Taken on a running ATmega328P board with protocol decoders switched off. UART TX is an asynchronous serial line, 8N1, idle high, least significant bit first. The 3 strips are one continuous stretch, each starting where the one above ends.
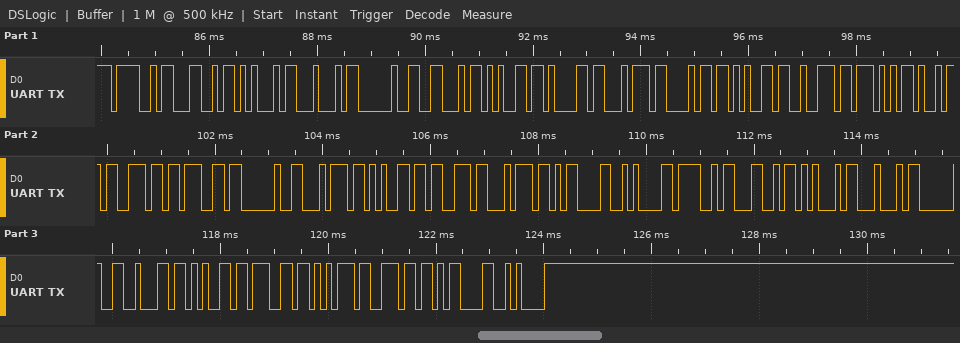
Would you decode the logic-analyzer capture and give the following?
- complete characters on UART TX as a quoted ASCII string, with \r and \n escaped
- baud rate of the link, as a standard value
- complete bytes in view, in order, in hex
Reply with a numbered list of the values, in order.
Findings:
1. "OLED FeatherWing test\r\nOLED begun\r\n"
2. 9600 baud
3. 4F 4C 45 44 20 46 65 61 74 68 65 72 57 69 6E 67 20 74 65 73 74 0D 0A 4F 4C 45 44 20 62 65 67 75 6E 0D 0A
